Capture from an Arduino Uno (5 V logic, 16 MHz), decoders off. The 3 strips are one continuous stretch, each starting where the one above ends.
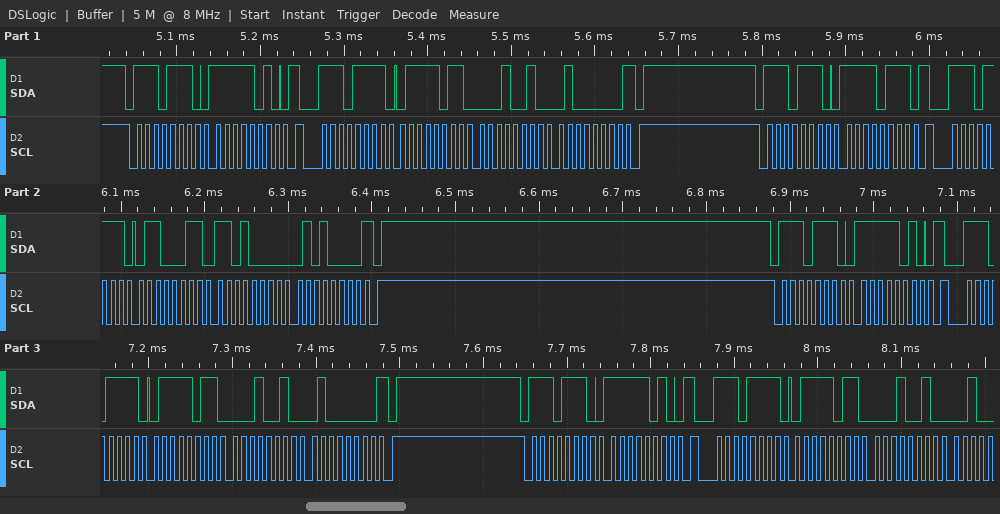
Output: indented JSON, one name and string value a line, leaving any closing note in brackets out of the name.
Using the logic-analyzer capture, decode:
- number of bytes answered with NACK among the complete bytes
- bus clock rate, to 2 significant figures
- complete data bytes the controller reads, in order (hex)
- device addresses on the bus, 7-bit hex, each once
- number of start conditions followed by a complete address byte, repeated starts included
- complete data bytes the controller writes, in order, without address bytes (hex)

{
  "number of bytes answered with NACK among the complete bytes": "3",
  "bus clock rate, to 2 significant figures": "100 kHz",
  "complete data bytes the controller reads, in order": "7B 12 40 63 D0 50 7B 12 40 7B 12",
  "device addresses on the bus, 7-bit hex, each once": "0x77",
  "number of start conditions followed by a complete address byte, repeated starts included": "8",
  "complete data bytes the controller writes, in order, without address bytes": "FA F7 FA FA"
}
